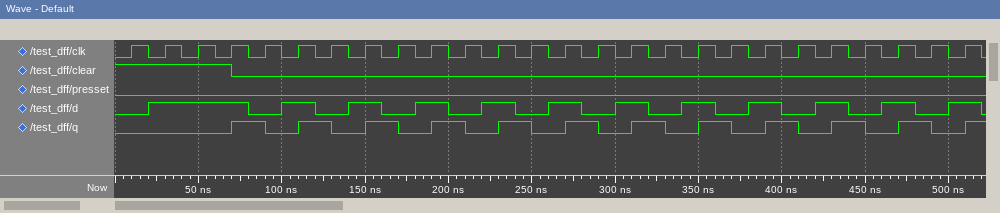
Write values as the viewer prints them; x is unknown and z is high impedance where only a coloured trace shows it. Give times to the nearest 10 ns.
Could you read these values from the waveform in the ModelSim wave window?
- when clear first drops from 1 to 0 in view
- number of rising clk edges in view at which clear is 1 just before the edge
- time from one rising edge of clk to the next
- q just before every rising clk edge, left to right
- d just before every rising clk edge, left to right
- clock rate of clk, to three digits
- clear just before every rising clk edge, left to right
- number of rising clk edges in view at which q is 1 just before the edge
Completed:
70 ns
4
20 ns
0 0 0 0 1 0 1 0 1 0 1 0 1 0 1 0 1 0 1 0 1 0 1 0 1 0
0 1 1 1 0 1 0 1 0 1 0 1 0 1 0 1 0 1 0 1 0 1 0 1 0 1
50.0 MHz
1 1 1 1 0 0 0 0 0 0 0 0 0 0 0 0 0 0 0 0 0 0 0 0 0 0
11
